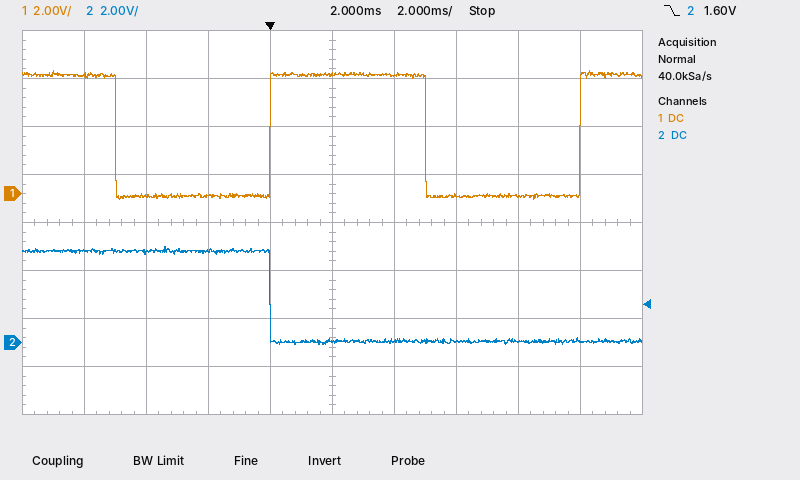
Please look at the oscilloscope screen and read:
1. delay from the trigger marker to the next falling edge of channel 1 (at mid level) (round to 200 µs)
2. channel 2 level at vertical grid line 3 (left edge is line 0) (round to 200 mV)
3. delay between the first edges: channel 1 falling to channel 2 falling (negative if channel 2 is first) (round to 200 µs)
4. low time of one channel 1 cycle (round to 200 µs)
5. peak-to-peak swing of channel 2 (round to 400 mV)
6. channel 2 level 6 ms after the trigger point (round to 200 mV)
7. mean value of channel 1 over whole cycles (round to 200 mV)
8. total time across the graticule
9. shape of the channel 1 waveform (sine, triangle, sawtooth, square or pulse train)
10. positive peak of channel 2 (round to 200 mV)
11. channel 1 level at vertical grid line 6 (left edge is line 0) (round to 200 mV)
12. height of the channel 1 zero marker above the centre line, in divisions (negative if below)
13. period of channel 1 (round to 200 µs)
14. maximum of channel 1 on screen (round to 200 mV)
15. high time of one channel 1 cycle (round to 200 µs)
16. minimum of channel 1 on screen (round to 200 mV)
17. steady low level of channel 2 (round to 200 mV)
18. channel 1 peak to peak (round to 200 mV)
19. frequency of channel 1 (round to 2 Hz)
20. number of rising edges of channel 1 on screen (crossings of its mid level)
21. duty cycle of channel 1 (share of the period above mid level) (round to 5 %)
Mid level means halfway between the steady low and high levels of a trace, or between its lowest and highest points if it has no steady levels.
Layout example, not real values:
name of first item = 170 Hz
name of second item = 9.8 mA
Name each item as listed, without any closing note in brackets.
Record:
delay from the trigger marker to the next falling edge of channel 1 (at mid level) = 5.0 ms
channel 2 level at vertical grid line 3 (left edge is line 0) = 3.8 V
delay between the first edges: channel 1 falling to channel 2 falling (negative if channel 2 is first) = +5.0 ms
low time of one channel 1 cycle = 5.0 ms
peak-to-peak swing of channel 2 = 4.0 V
channel 2 level 6 ms after the trigger point = 0.0 V
mean value of channel 1 over whole cycles = 2.4 V
total time across the graticule = 20 ms
shape of the channel 1 waveform = square
positive peak of channel 2 = 4.0 V
channel 1 level at vertical grid line 6 (left edge is line 0) = 5.0 V
height of the channel 1 zero marker above the centre line, in divisions = +0.6 div
period of channel 1 = 10.0 ms
maximum of channel 1 on screen = 5.2 V
high time of one channel 1 cycle = 5.0 ms
minimum of channel 1 on screen = -200 mV
steady low level of channel 2 = 0.0 V
channel 1 peak to peak = 5.4 V
frequency of channel 1 = 100 Hz
number of rising edges of channel 1 on screen = 2
duty cycle of channel 1 (share of the period above mid level) = 50 %
